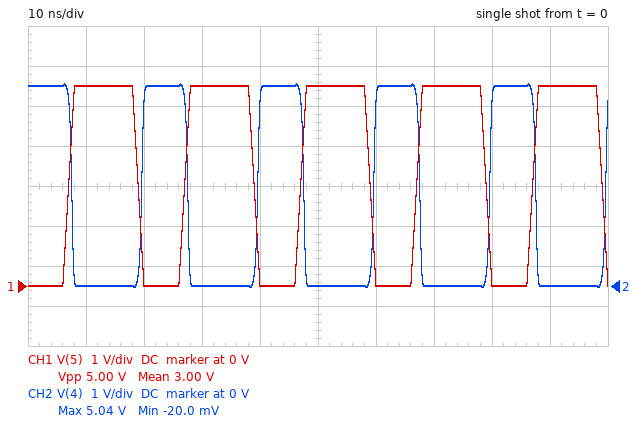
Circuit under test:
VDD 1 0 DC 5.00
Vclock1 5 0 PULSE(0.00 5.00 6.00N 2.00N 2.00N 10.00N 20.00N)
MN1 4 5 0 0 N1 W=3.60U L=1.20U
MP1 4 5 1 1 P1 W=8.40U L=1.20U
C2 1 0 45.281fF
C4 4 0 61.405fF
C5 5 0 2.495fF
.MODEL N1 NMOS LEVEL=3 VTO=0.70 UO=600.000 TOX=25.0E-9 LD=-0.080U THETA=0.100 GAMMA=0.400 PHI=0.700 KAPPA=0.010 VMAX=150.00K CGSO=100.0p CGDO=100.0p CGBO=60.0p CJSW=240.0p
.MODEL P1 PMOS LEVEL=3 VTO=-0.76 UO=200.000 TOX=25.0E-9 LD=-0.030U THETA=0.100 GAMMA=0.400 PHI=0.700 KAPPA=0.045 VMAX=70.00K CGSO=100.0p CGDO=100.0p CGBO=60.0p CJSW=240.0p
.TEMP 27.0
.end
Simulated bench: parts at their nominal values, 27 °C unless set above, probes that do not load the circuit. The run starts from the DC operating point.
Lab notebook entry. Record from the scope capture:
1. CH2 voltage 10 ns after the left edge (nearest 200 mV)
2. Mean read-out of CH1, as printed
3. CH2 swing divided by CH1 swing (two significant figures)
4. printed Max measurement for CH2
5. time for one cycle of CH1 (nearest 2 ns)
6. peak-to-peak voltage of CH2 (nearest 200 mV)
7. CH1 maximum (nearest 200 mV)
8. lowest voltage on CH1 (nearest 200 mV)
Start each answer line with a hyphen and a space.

- 0 V
- 3.00 V
- 1.0
- 5.04 V
- 20 ns
- 5.0 V
- 5.0 V
- 0 V
